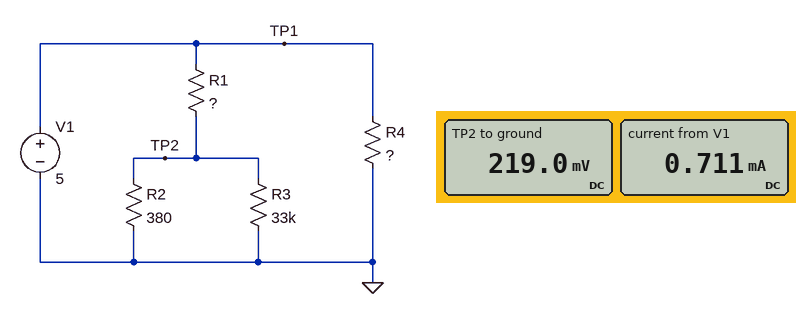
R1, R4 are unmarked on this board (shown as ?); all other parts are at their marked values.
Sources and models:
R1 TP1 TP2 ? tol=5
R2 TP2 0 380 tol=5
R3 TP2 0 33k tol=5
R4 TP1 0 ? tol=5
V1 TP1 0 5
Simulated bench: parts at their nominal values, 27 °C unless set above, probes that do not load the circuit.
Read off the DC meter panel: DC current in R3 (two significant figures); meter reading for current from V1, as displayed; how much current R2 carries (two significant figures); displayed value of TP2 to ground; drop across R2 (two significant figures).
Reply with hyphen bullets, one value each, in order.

- 6.6 µA
- 0.711 mA
- 580 µA
- 219.0 mV
- 220 mV
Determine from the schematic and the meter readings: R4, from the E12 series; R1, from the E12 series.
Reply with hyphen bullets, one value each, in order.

- 39 kΩ
- 8.2 kΩ
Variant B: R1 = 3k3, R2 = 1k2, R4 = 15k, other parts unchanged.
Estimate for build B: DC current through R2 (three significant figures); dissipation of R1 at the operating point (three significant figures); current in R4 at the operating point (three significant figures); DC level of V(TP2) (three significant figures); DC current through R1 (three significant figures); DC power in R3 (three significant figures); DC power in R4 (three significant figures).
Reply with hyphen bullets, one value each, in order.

- 1.08 mA
- 4.15 mW
- 333 µA
- 1.30 V
- 1.12 mA
- 51.1 µW
- 1.67 mW
